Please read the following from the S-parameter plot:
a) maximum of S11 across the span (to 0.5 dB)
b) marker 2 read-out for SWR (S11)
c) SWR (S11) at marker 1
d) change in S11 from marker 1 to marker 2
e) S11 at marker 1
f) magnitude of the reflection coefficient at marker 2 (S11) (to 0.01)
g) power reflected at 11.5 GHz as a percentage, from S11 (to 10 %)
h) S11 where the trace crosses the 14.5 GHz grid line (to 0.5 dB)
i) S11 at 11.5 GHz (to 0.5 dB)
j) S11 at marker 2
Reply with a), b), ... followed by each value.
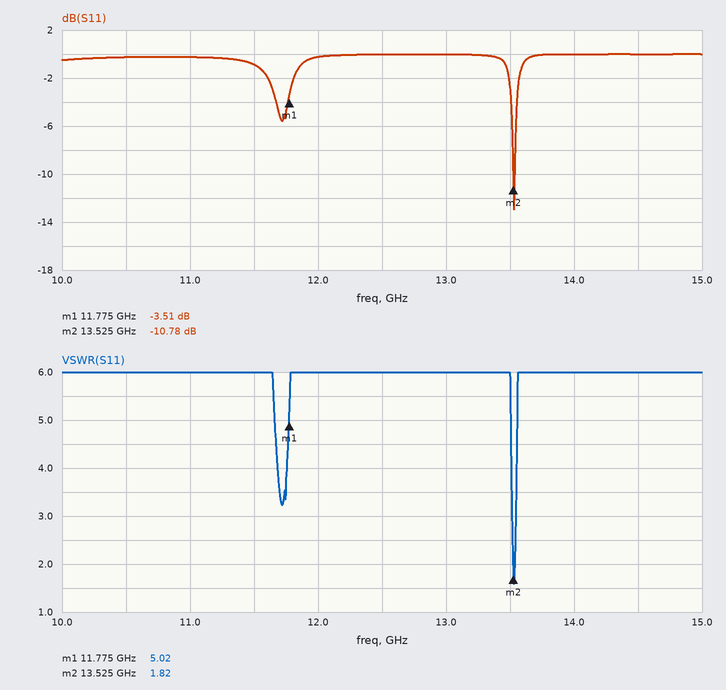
a) 0.0 dB
b) 1.82
c) 5.02
d) -7.27 dB
e) -3.51 dB
f) 0.29
g) 80 %
h) 0.0 dB
i) -1.0 dB
j) -10.78 dB
